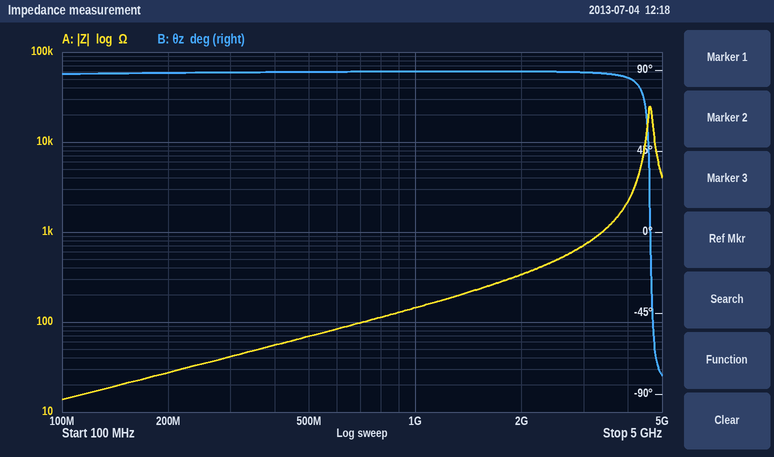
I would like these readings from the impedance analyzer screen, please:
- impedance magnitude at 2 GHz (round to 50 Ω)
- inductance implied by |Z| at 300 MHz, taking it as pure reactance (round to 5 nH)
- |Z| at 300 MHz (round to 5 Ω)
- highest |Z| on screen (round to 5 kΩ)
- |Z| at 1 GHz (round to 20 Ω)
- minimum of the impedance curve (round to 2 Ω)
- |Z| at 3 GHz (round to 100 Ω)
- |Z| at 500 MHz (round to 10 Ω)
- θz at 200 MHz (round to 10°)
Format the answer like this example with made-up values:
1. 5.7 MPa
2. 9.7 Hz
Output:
1. 350 Ω
2. 20 nH
3. 40 Ω
4. 25 kΩ
5. 140 Ω
6. 14 Ω
7. 700 Ω
8. 70 Ω
9. 90°
